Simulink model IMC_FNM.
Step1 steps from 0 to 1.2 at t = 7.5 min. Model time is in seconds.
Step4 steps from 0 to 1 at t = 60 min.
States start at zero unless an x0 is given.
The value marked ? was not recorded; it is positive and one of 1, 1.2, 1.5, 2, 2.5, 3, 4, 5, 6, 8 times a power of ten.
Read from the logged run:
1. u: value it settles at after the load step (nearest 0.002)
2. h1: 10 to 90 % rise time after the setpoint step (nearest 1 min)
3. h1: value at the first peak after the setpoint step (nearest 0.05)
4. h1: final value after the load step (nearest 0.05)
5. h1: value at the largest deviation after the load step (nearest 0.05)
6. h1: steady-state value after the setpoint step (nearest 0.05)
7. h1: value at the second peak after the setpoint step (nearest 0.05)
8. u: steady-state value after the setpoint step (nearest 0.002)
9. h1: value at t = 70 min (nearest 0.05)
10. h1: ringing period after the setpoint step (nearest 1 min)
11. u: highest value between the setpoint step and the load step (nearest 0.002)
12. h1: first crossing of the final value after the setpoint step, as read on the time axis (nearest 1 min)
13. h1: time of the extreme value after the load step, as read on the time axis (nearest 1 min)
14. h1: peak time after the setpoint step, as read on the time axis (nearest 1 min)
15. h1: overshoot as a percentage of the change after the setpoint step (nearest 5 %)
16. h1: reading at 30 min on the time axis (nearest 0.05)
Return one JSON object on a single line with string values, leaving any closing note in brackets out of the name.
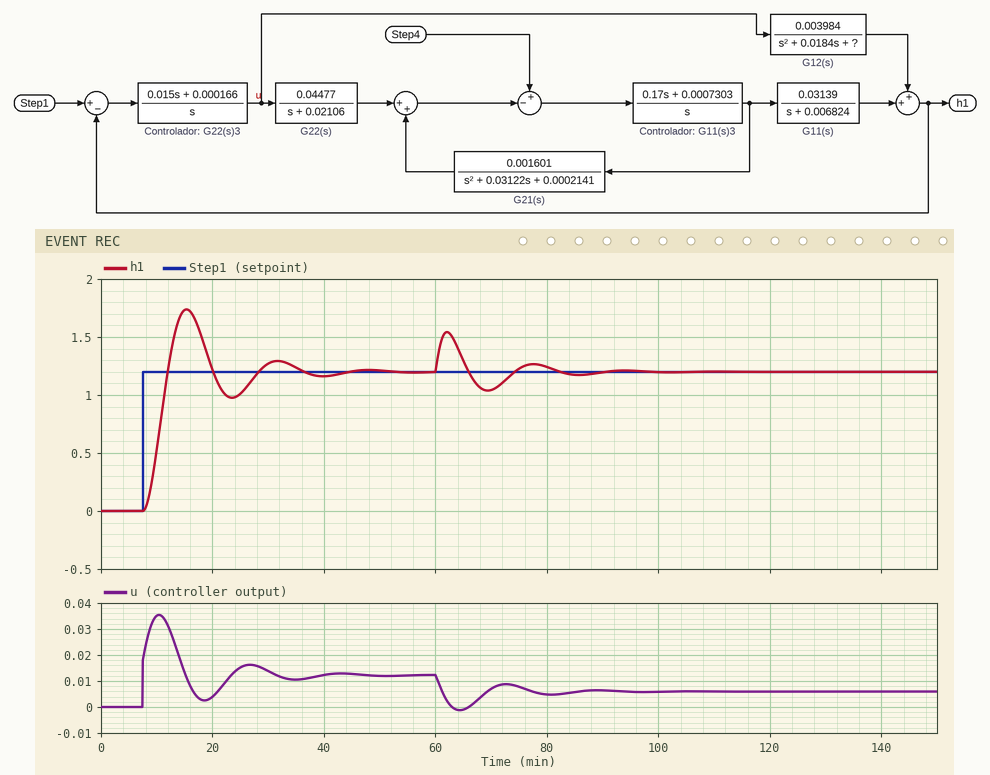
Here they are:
{"u: value it settles at after the load step": "0.006", "h1: 10 to 90 % rise time after the setpoint step": "3 min", "h1: value at the first peak after the setpoint step": "1.75", "h1: final value after the load step": "1.20", "h1: value at the largest deviation after the load step": "1.55", "h1: steady-state value after the setpoint step": "1.20", "h1: value at the second peak after the setpoint step": "1.30", "u: steady-state value after the setpoint step": "0.012", "h1: value at t = 70 min": "1.05", "h1: ringing period after the setpoint step": "16 min", "u: highest value between the setpoint step and the load step": "0.036", "h1: first crossing of the final value after the setpoint step, as read on the time axis": "12 min", "h1: time of the extreme value after the load step, as read on the time axis": "62 min", "h1: peak time after the setpoint step, as read on the time axis": "15 min", "h1: overshoot as a percentage of the change after the setpoint step": "45 %", "h1: reading at 30 min on the time axis": "1.25"}
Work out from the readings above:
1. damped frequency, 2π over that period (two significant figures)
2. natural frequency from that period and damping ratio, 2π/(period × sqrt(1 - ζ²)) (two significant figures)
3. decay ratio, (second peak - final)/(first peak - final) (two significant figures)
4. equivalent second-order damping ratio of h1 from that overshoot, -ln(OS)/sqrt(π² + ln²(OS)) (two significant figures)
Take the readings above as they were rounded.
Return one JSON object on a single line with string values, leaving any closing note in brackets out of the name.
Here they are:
{"damped frequency, 2π over that period": "0.39 rad/min", "natural frequency from that period and damping ratio, 2π/(period × sqrt(1 - ζ²))": "0.41 rad/min", "decay ratio, (second peak - final)/(first peak - final)": "0.18", "equivalent second-order damping ratio of h1 from that overshoot, -ln(OS)/sqrt(π² + ln²(OS))": "0.25"}
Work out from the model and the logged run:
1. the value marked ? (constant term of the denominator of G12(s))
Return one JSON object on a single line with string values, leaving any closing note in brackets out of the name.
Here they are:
{"the value marked ? (constant term of the denominator of G12(s))": "4e-05"}
